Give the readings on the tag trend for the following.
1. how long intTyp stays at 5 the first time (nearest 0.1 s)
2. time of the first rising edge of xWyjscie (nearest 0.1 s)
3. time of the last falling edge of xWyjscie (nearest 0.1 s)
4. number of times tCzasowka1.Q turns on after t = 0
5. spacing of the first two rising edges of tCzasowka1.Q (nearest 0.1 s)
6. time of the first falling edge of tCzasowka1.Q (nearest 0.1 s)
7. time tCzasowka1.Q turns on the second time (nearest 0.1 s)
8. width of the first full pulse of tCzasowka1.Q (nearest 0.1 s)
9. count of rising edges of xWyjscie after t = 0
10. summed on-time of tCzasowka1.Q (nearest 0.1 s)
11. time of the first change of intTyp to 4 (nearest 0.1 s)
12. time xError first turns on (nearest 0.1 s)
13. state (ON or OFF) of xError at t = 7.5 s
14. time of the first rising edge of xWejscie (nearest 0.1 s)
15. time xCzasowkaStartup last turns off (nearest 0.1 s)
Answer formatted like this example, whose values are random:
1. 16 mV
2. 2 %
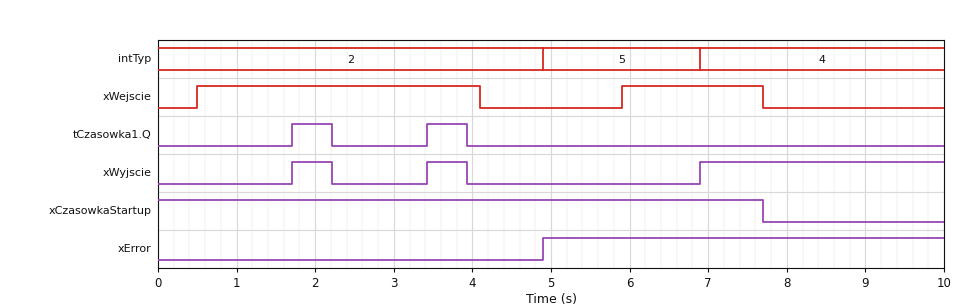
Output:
1. 2.0 s
2. 1.7 s
3. 3.9 s
4. 2
5. 1.7 s
6. 2.2 s
7. 3.4 s
8. 0.5 s
9. 3
10. 1.0 s
11. 6.9 s
12. 4.9 s
13. ON
14. 0.5 s
15. 7.7 s
